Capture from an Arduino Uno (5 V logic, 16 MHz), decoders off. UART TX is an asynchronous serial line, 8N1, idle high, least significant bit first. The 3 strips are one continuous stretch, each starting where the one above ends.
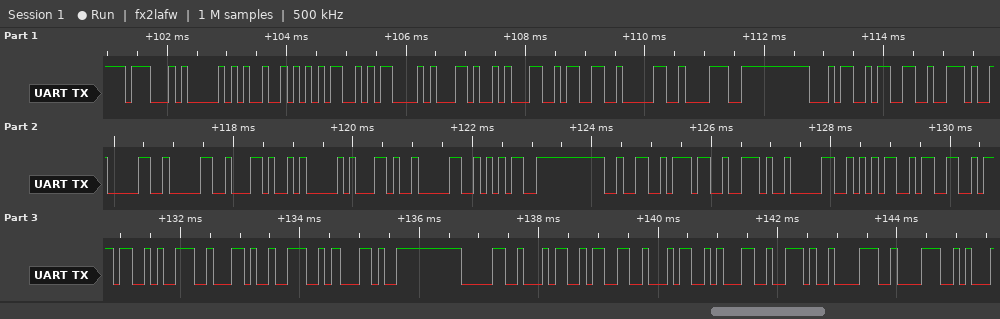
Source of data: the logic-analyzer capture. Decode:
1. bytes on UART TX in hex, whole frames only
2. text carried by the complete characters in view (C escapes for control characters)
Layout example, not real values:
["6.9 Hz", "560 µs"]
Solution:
["47 50 52 4D 43 2C 31 33 30 38 34 33 2E 30 30 2C 41 2C 30 35 32 37 2E 30 35 33 37 39 2C 4E 2C 30 34 33 34 31 2E 38 38", "\"GPRMC,130843.00,A,0527.05379,N,04341.88\""]
